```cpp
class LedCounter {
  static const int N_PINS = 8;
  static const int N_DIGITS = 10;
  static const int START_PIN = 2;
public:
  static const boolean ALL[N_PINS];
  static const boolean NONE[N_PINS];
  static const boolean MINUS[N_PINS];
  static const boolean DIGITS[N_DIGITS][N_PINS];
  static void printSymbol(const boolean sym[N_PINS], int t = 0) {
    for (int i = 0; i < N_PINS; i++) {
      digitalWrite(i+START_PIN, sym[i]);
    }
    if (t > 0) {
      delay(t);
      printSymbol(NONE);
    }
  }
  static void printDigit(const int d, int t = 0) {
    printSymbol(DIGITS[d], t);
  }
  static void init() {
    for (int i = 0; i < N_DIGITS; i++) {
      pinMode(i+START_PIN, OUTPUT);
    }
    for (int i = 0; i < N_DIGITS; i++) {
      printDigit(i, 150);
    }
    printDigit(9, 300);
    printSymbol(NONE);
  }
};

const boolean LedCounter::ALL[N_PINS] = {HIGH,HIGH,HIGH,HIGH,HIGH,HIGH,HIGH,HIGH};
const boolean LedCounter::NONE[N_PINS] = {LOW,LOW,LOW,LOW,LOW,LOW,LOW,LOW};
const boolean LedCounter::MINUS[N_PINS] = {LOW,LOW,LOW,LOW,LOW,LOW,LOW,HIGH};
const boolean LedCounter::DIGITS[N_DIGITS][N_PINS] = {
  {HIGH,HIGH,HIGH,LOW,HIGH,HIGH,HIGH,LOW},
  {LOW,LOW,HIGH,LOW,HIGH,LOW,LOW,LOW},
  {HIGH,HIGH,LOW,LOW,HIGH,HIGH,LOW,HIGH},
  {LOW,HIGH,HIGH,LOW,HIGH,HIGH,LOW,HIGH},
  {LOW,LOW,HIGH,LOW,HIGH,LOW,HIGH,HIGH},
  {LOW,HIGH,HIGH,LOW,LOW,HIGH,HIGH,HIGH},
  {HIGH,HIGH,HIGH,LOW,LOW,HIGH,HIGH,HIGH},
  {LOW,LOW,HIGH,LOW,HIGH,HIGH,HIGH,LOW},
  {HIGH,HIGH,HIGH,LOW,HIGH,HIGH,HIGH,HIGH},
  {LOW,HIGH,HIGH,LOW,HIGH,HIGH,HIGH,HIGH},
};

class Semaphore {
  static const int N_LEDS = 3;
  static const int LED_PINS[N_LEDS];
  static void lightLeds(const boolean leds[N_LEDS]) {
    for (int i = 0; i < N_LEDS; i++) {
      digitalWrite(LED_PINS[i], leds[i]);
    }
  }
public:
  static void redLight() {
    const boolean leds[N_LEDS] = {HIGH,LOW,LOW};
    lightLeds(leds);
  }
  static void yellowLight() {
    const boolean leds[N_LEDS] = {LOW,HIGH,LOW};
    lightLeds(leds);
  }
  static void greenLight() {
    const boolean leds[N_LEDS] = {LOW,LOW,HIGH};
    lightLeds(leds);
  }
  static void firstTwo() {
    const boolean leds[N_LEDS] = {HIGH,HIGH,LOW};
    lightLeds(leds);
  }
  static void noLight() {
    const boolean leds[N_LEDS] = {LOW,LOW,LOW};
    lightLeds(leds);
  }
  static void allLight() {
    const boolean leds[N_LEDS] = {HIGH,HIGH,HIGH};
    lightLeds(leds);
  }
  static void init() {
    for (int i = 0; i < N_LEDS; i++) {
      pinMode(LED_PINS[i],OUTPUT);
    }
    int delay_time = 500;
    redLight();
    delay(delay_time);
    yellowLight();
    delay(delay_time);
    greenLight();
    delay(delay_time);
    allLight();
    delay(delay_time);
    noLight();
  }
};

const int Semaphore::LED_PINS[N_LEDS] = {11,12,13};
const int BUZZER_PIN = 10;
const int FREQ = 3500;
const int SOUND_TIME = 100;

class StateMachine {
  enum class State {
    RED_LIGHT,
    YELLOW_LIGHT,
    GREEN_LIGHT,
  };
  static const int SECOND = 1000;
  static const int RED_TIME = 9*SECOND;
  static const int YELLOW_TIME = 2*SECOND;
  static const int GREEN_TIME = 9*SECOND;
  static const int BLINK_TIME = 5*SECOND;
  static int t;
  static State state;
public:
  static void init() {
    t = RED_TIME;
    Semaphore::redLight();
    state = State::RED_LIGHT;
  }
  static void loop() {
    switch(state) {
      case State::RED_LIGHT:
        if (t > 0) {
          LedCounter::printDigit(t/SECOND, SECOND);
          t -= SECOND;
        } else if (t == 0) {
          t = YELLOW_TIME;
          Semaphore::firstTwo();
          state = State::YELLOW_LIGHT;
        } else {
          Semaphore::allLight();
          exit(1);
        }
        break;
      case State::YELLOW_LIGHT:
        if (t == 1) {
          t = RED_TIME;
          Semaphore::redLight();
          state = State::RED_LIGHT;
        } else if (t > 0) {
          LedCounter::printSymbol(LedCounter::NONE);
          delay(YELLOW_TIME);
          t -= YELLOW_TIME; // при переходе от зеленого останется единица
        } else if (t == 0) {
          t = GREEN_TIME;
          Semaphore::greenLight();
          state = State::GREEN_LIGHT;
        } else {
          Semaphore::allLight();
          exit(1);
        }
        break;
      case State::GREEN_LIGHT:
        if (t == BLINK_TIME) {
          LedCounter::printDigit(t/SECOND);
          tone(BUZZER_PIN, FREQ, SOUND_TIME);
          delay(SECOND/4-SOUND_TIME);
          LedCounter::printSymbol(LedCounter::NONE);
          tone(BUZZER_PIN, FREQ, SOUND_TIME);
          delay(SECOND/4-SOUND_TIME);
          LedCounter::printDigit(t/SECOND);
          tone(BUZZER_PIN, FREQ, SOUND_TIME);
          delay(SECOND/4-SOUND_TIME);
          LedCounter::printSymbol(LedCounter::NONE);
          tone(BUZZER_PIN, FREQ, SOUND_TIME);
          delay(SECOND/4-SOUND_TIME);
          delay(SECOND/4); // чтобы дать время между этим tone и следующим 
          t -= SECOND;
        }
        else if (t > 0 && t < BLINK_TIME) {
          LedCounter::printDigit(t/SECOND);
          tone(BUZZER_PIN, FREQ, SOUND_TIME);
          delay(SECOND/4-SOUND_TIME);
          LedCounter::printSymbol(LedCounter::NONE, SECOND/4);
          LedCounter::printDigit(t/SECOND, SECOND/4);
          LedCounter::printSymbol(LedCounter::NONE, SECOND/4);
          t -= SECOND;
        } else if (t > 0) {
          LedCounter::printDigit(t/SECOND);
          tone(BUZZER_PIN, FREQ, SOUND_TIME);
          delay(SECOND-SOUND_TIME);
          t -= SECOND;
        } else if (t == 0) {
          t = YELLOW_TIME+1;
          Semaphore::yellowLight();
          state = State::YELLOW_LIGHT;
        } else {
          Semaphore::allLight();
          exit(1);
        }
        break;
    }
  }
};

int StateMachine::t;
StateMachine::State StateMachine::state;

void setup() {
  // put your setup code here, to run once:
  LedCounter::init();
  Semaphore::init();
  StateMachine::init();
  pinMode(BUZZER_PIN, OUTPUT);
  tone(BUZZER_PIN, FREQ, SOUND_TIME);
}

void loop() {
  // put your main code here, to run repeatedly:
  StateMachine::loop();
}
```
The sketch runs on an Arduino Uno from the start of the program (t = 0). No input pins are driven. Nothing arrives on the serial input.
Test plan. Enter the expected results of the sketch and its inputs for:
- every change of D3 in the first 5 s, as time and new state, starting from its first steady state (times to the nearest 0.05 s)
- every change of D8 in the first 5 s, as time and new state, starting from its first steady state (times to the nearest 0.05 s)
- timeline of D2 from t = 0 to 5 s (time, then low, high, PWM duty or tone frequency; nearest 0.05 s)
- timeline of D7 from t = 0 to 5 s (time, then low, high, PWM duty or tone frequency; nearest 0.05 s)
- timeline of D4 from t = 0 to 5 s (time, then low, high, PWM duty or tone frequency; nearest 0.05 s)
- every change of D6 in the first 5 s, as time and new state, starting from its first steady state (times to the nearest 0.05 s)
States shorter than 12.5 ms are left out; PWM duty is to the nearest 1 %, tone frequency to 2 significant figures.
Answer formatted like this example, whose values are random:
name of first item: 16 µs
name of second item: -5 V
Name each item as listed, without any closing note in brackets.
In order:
every change of D3 in the first 5 s, as time and new state, starting from its first steady state: 0 s high; 0.15 s low; 0.3 s high; 0.6 s low; 0.75 s high; 1.05 s low; 1.2 s high; 1.8 s low; 3.8 s high
every change of D8 in the first 5 s, as time and new state, starting from its first steady state: 0 s high; 0.15 s low; 0.6 s high; 1.8 s low; 3.8 s high
timeline of D2 from t = 0 to 5 s: 0 s high; 0.15 s low; 0.3 s high; 0.45 s low; 0.9 s high; 1.05 s low; 1.2 s high; 1.35 s low; 4.8 s high
timeline of D7 from t = 0 to 5 s: 0 s high; 0.15 s low; 0.3 s high; 0.6 s low; 0.75 s high; 1.8 s low; 3.8 s high
timeline of D4 from t = 0 to 5 s: 0 s high; 0.3 s low; 0.45 s high; 1.8 s low; 3.8 s high
every change of D6 in the first 5 s, as time and new state, starting from its first steady state: 0 s high; 0.75 s low; 1.05 s high; 1.8 s low; 3.8 s high
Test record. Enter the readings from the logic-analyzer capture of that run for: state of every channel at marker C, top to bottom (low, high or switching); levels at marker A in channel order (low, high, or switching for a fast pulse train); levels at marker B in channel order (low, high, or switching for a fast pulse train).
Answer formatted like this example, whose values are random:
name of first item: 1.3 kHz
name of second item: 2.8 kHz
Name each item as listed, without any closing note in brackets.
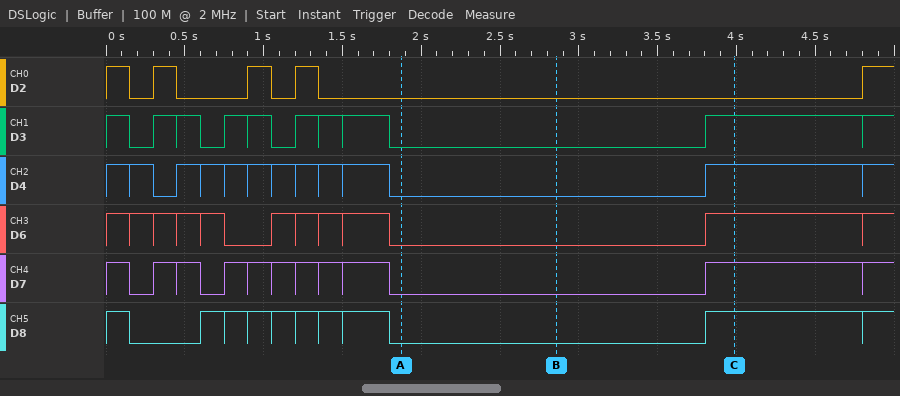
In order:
state of every channel at marker C, top to bottom: D2 low, D3 high, D4 high, D6 high, D7 high, D8 high
levels at marker A in channel order: D2 low, D3 low, D4 low, D6 low, D7 low, D8 low
levels at marker B in channel order: D2 low, D3 low, D4 low, D6 low, D7 low, D8 low
